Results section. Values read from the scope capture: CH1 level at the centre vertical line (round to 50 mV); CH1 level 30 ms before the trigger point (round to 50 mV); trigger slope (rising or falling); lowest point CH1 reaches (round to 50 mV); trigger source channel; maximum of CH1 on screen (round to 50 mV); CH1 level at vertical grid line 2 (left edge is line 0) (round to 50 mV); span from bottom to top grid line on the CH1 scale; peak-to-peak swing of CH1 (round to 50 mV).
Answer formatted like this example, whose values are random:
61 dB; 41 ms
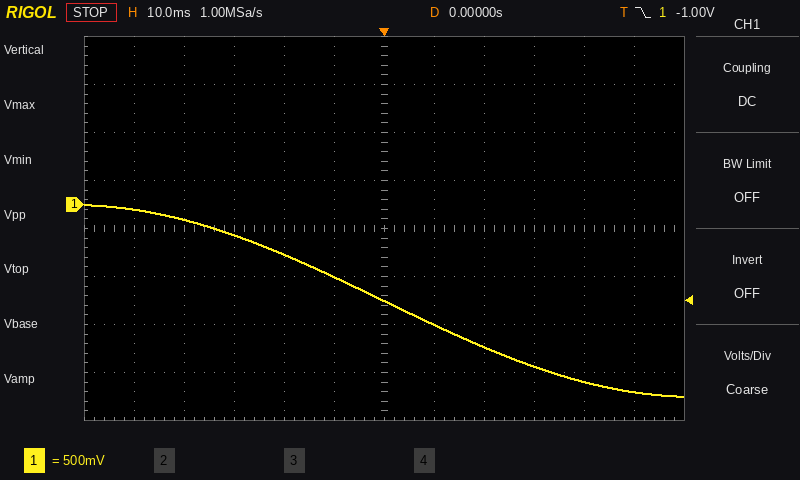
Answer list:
-1.00 V; -300 mV; falling; -2.00 V; CH1; 0 mV; -150 mV; 4 V; 2.00 V
